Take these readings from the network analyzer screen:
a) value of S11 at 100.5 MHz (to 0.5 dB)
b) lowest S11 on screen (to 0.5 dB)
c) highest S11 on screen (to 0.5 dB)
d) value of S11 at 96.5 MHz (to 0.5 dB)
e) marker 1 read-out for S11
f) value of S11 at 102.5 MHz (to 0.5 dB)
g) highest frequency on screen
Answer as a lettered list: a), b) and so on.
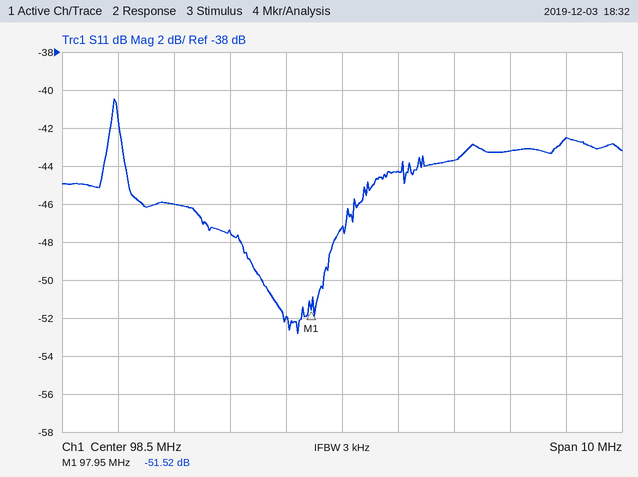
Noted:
a) -43.5 dB
b) -53.0 dB
c) -40.5 dB
d) -47.5 dB
e) -51.52 dB
f) -42.5 dB
g) 103.5 MHz
